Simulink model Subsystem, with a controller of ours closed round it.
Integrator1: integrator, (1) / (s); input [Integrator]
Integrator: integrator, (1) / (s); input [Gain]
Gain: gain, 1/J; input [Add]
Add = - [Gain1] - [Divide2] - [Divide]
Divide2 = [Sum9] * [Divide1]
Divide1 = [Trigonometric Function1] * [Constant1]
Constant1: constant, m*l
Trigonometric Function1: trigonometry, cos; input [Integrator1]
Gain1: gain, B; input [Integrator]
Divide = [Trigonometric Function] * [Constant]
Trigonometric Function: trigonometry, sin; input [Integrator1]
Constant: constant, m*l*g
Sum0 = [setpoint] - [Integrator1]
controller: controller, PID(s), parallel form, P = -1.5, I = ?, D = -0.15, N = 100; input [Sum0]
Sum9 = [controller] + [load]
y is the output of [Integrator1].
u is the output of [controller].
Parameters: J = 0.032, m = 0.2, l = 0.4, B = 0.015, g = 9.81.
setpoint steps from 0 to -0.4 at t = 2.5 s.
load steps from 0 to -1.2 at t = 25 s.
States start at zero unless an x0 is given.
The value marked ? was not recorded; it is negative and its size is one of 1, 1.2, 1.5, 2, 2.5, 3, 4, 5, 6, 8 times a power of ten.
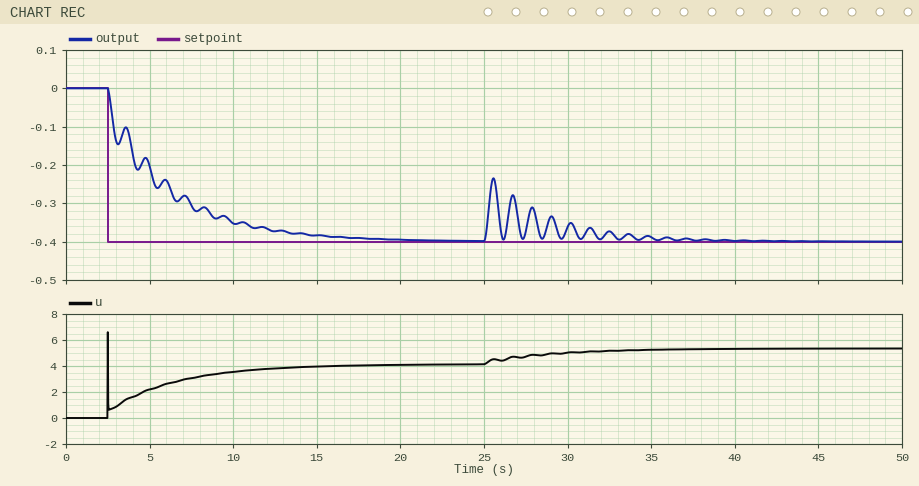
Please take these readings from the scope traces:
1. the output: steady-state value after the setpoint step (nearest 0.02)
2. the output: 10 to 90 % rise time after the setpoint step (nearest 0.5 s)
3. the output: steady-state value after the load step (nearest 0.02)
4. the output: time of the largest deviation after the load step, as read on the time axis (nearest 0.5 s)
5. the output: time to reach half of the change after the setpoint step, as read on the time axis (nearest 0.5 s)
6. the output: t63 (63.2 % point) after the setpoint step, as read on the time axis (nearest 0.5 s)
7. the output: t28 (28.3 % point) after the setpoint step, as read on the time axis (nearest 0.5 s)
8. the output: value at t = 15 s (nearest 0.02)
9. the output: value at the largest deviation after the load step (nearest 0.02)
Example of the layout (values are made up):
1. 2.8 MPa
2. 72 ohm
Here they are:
1. -0.40
2. 8.5 s
3. -0.40
4. 25.5 s
5. 4.0 s
6. 5.5 s
7. 3.0 s
8. -0.38
9. -0.24
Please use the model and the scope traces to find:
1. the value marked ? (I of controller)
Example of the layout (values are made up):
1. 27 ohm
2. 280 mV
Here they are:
1. -3
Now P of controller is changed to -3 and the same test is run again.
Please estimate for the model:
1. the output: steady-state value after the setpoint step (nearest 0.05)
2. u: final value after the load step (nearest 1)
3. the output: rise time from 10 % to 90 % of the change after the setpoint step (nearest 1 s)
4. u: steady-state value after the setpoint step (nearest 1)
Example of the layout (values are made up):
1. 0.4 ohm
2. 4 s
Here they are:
1. -0.40
2. 5
3. 9 s
4. 4
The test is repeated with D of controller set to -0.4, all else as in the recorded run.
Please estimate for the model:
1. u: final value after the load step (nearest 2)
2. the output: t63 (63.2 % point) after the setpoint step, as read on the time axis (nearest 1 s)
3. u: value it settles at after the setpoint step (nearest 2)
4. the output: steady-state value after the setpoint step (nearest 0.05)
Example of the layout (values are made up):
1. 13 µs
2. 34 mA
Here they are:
1. 6
2. 6 s
3. 4
4. -0.40
